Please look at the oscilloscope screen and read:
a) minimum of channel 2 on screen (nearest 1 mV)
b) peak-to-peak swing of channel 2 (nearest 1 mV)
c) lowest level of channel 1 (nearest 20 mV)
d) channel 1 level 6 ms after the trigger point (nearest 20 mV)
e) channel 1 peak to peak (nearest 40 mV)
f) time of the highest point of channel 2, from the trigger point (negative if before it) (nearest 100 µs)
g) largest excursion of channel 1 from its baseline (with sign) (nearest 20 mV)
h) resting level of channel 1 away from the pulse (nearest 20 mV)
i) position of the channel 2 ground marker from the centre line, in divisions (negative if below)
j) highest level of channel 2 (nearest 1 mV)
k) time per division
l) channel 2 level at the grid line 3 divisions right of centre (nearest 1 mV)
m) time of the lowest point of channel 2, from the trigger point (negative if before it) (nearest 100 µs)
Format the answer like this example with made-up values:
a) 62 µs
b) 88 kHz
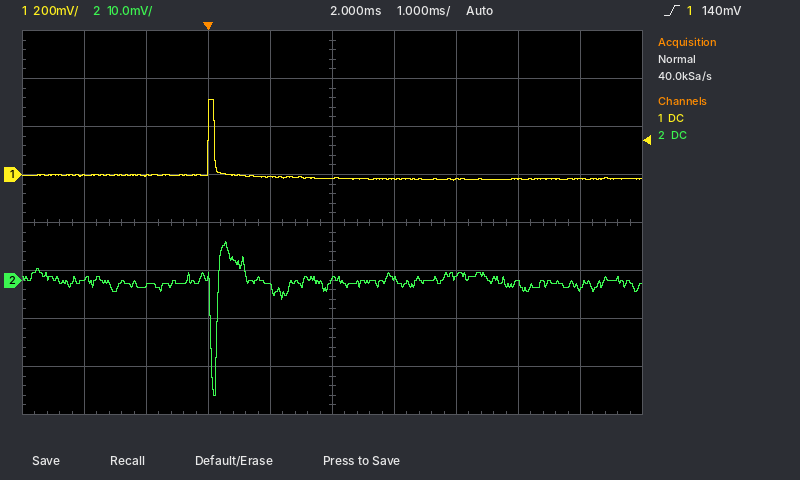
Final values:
a) -24 mV
b) 32 mV
c) -20 mV
d) -20 mV
e) 320 mV
f) +300 µs
g) +320 mV
h) -20 mV
i) -1.2 div
j) 8 mV
k) 1 ms
l) -1 mV
m) +100 µs
